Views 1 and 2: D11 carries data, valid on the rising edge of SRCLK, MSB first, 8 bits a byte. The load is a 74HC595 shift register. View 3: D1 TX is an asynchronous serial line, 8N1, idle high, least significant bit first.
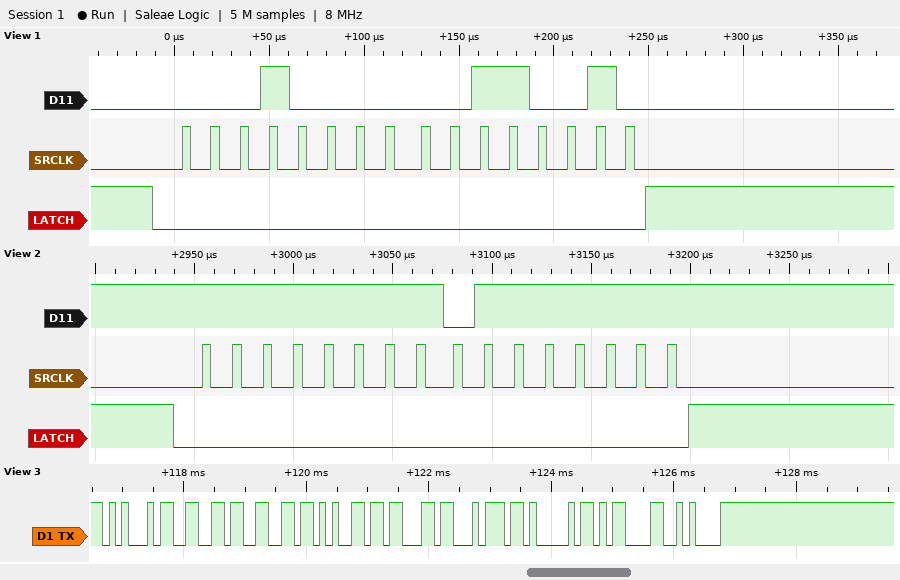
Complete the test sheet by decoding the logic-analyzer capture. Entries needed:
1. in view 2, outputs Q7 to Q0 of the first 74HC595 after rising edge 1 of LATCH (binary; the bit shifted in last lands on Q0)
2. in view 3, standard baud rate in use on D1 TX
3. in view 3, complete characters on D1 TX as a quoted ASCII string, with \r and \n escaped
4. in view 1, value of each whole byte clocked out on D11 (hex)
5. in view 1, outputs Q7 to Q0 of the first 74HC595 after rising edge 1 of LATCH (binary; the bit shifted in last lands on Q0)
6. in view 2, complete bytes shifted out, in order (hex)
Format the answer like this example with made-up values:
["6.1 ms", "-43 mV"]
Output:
["01111111", "9600 baud", "\"EffectA\\r\\n\"", "0x10 0x32", "00110010", "0xFF 0x7F"]
